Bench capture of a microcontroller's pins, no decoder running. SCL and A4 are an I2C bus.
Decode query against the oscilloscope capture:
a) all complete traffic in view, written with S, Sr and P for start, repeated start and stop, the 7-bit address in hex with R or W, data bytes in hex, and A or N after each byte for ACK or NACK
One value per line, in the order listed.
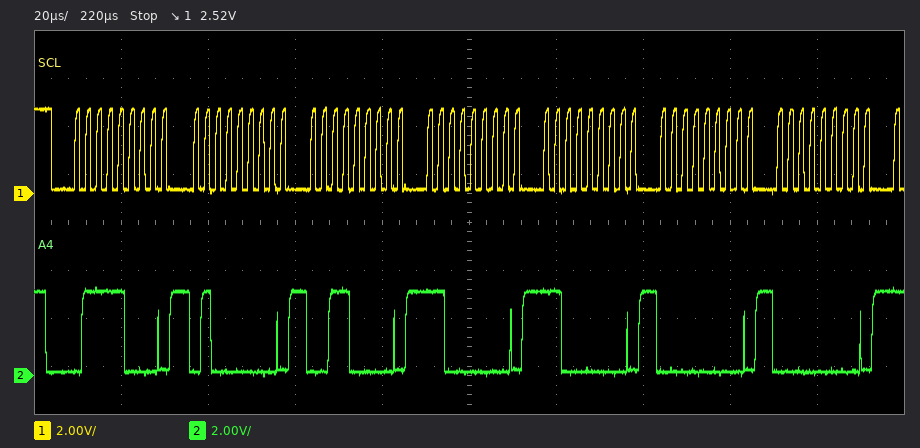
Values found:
S 3CW A 40 A 30 A C0 A C0 A 00 A 00 A
